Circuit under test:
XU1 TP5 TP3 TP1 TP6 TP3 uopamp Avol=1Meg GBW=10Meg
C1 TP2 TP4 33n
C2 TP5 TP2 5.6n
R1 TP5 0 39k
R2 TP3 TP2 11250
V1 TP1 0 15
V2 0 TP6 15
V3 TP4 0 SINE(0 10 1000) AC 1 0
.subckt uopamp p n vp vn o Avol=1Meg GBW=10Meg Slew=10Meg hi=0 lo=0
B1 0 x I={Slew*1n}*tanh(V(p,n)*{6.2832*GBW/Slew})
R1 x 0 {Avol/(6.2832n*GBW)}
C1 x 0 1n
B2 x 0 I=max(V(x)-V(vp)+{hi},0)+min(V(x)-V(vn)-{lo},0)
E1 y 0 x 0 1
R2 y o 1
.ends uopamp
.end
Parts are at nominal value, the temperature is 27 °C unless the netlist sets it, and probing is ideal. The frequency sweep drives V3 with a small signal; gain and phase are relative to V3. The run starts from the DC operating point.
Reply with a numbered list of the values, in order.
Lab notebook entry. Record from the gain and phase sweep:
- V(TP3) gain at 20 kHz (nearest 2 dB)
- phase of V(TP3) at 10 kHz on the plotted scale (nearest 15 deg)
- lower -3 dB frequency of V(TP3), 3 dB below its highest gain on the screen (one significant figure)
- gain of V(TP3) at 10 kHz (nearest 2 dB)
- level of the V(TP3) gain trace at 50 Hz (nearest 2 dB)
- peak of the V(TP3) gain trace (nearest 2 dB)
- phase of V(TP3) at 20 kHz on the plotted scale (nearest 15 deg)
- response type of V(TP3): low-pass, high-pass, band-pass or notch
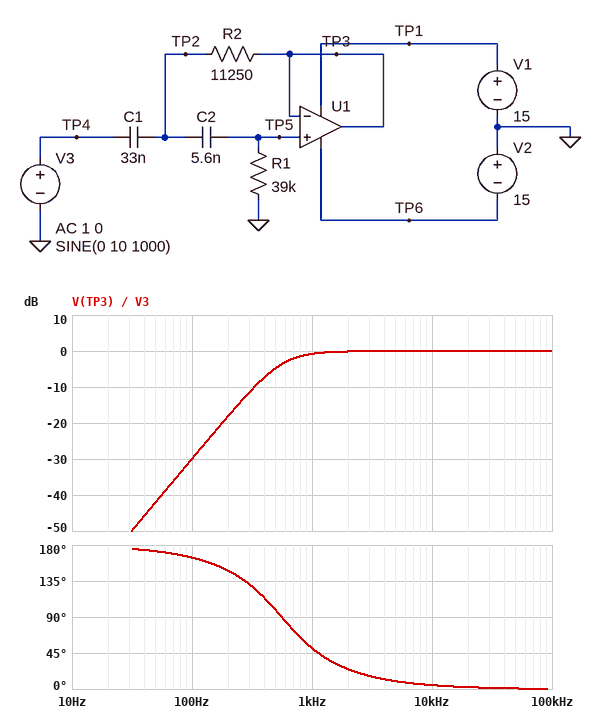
1. 0 dB
2. 0 deg
3. 600 Hz
4. 0 dB
5. -42 dB
6. 0 dB
7. 0 deg
8. high-pass
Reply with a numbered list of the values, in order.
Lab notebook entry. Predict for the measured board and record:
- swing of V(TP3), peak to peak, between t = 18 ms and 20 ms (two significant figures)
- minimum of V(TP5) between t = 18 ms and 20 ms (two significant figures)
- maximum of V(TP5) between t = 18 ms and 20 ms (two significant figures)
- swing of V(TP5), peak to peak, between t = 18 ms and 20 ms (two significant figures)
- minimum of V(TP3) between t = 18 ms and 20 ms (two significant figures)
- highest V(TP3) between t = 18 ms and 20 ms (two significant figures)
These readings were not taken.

1. 18 V
2. -9.1 V
3. 9.1 V
4. 18 V
5. -9.1 V
6. 9.1 V
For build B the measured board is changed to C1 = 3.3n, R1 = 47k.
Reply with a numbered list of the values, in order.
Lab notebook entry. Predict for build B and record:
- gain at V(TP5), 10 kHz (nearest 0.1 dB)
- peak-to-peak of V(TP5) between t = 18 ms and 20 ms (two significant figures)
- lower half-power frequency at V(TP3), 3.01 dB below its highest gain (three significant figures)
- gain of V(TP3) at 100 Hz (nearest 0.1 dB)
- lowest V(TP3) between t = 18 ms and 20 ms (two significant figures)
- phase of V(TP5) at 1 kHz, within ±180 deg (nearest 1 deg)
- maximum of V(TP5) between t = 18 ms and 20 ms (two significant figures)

1. 0.1 dB
2. 8.8 V
3. 1.38 kHz
4. -48.3 dB
5. -4.4 V
6. 134 deg
7. 4.4 V
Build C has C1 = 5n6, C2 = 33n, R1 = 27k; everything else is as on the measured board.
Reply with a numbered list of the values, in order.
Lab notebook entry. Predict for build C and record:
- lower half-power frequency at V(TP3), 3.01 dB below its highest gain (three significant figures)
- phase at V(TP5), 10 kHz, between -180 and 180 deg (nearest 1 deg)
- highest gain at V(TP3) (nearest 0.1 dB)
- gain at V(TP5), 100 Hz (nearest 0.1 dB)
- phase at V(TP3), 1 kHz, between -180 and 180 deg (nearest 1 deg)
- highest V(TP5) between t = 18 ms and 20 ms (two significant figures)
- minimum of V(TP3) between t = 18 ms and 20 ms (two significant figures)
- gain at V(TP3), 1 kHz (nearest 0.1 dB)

1. 923 Hz
2. 7 deg
3. 0 dB
4. -33.2 dB
5. 66 deg
6. 7.4 V
7. -7.4 V
8. -2.6 dB
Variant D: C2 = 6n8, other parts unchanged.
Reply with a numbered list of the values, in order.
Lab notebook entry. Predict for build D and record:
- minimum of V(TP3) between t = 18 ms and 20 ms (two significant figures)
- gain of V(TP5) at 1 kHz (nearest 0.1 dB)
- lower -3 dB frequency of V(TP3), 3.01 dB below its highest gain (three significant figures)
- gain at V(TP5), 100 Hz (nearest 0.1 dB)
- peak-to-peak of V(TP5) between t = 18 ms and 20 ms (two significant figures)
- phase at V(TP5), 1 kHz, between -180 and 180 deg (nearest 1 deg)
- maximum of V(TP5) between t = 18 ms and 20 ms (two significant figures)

1. -9.6 V
2. -0.3 dB
3. 512 Hz
4. -28.2 dB
5. 19 V
6. 44 deg
7. 9.6 V
